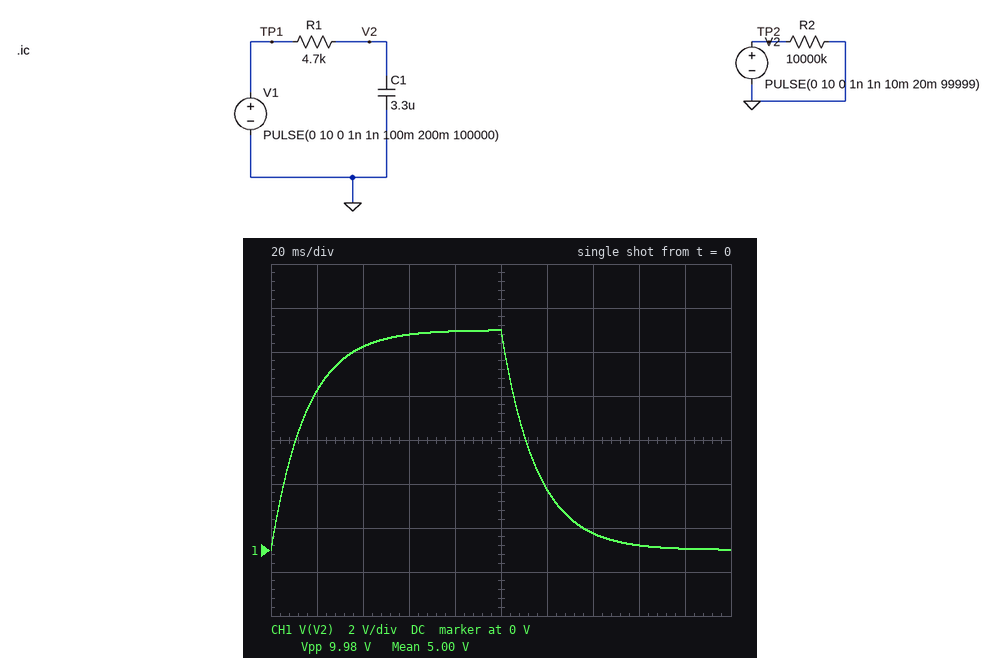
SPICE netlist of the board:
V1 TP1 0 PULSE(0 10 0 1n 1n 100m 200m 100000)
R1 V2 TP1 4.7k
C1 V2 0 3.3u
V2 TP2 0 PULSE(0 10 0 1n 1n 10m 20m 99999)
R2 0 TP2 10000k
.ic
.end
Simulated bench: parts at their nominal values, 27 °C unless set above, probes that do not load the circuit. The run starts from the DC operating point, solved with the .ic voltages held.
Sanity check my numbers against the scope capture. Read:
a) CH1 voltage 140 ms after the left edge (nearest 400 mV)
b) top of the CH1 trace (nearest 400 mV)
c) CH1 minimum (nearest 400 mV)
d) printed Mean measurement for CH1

800 mV
10.0 V
0 V
5.00 V
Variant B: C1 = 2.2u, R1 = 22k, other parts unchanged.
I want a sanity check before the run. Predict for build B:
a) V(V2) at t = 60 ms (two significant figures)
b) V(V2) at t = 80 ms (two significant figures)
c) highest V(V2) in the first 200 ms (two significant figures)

7.1 V
8.1 V
8.7 V
